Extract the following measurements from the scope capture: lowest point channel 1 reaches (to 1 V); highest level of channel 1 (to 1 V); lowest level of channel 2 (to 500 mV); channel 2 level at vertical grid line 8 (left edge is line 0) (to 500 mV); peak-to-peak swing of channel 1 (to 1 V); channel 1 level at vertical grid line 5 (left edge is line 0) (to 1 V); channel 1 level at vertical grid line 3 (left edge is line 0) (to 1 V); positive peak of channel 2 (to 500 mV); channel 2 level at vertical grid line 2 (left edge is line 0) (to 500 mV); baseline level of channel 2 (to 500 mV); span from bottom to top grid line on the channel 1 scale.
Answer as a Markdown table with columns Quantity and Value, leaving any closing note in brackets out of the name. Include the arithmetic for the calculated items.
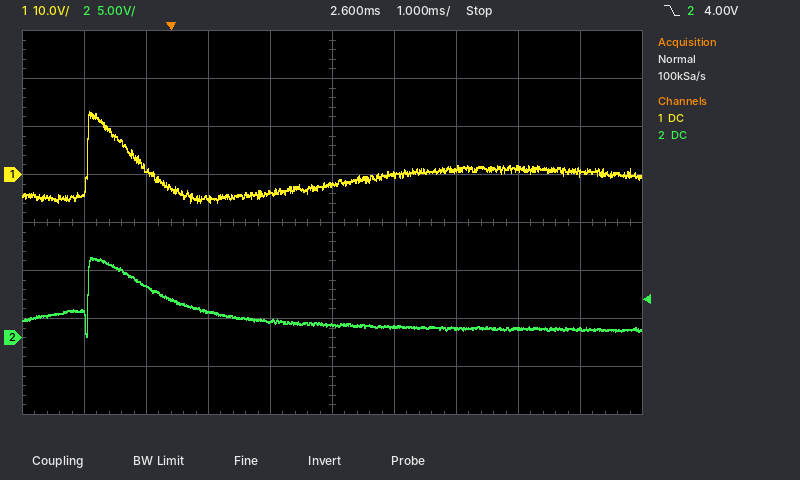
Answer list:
| Quantity | Value |
|---|---|
| lowest point channel 1 reaches | -6 V |
| highest level of channel 1 | 13 V |
| lowest level of channel 2 | 0.0 V |
| channel 2 level at vertical grid line 8 (left edge is line 0) | 1.0 V |
| peak-to-peak swing of channel 1 | 13 V − (-6 V) = 19 V |
| channel 1 level at vertical grid line 5 (left edge is line 0) | -2 V |
| channel 1 level at vertical grid line 3 (left edge is line 0) | -5 V |
| positive peak of channel 2 | 8.5 V |
| channel 2 level at vertical grid line 2 (left edge is line 0) | 5.5 V |
| baseline level of channel 2 | 1.0 V |
| span from bottom to top grid line on the channel 1 scale | 80 V |
